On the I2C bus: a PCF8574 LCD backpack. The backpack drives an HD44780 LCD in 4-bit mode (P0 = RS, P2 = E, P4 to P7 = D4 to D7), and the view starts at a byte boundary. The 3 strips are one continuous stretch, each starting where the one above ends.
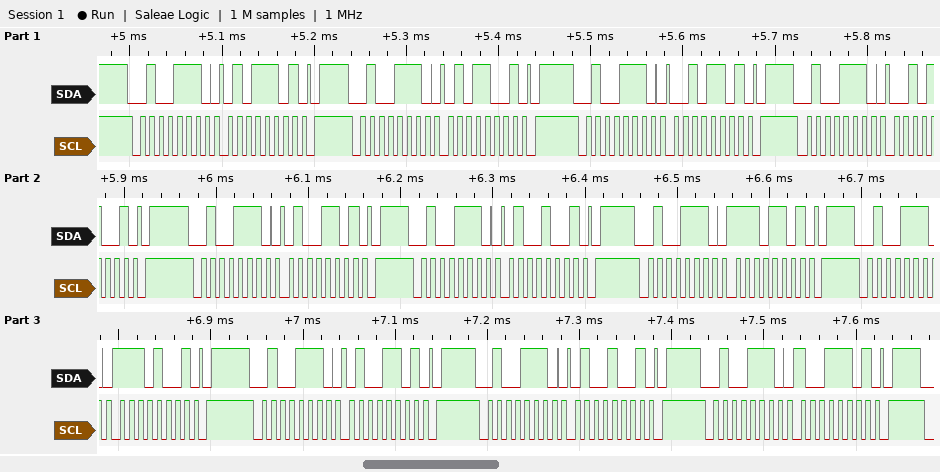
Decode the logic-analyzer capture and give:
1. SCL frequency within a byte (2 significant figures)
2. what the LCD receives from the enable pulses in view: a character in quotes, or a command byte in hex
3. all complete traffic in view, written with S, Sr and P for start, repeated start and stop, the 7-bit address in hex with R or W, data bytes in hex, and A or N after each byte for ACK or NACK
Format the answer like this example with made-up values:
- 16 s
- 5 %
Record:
- 100 kHz
- 'R' 'N'
- S 27W A 5D A P S 27W A 59 A P S 27W A 2D A P S 27W A 29 A P S 27W A 4D A P S 27W A 49 A P S 27W A ED A P S 27W A E9 A P S 27W A 4D A P S 27W A 49 A P S 27W A 9D A P
